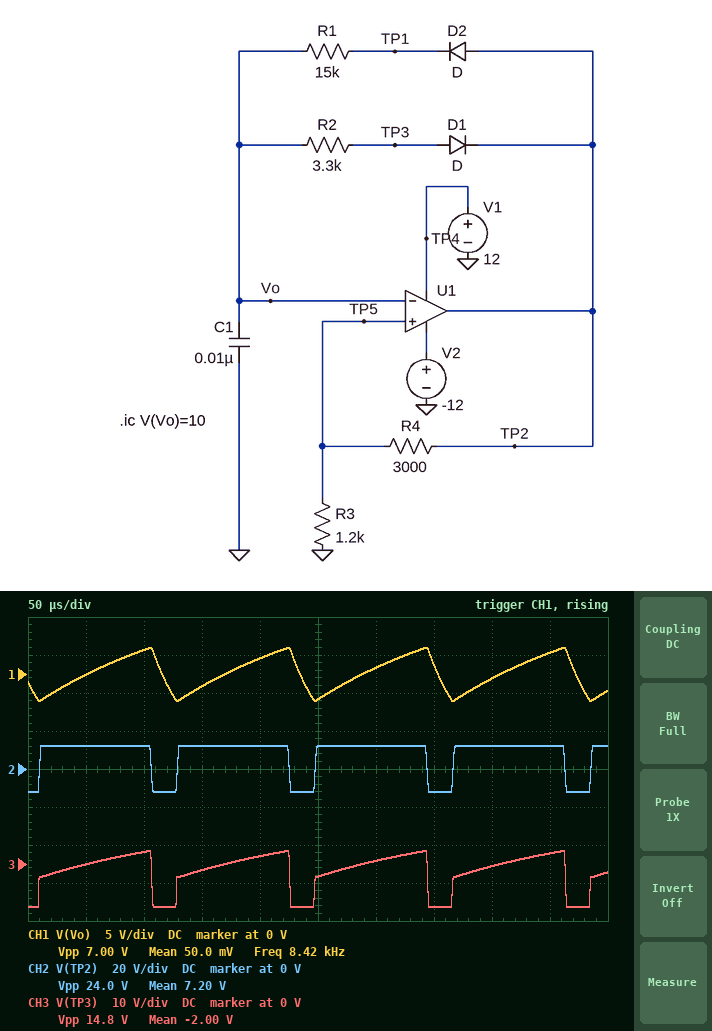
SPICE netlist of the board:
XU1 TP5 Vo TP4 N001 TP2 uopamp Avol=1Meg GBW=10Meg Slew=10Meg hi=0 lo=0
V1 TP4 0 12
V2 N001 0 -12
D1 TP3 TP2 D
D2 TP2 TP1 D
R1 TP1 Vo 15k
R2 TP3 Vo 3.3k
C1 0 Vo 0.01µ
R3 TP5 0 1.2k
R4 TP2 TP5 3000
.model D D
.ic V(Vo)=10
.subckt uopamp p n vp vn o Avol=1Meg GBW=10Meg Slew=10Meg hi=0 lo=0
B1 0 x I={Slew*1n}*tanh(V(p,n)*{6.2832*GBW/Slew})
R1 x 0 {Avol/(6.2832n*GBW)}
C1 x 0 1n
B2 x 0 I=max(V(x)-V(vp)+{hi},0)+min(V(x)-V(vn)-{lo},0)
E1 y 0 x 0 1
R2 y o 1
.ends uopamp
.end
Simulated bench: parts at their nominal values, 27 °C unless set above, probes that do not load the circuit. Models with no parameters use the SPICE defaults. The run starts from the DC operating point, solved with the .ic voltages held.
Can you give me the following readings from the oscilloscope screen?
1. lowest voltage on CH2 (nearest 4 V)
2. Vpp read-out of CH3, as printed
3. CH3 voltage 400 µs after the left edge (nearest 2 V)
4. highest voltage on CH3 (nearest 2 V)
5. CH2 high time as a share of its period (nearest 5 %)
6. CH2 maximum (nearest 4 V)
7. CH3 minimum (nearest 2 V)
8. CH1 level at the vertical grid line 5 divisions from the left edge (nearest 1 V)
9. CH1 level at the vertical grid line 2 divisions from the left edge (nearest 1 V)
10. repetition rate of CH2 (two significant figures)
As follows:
-12 V
14.8 V
0 V
4 V
80 %
12 V
-12 V
-3 V
3 V
8.4 kHz
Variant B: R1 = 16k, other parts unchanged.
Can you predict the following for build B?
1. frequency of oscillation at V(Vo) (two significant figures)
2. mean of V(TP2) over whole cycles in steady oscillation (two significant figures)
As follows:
8.0 kHz
7.7 V
